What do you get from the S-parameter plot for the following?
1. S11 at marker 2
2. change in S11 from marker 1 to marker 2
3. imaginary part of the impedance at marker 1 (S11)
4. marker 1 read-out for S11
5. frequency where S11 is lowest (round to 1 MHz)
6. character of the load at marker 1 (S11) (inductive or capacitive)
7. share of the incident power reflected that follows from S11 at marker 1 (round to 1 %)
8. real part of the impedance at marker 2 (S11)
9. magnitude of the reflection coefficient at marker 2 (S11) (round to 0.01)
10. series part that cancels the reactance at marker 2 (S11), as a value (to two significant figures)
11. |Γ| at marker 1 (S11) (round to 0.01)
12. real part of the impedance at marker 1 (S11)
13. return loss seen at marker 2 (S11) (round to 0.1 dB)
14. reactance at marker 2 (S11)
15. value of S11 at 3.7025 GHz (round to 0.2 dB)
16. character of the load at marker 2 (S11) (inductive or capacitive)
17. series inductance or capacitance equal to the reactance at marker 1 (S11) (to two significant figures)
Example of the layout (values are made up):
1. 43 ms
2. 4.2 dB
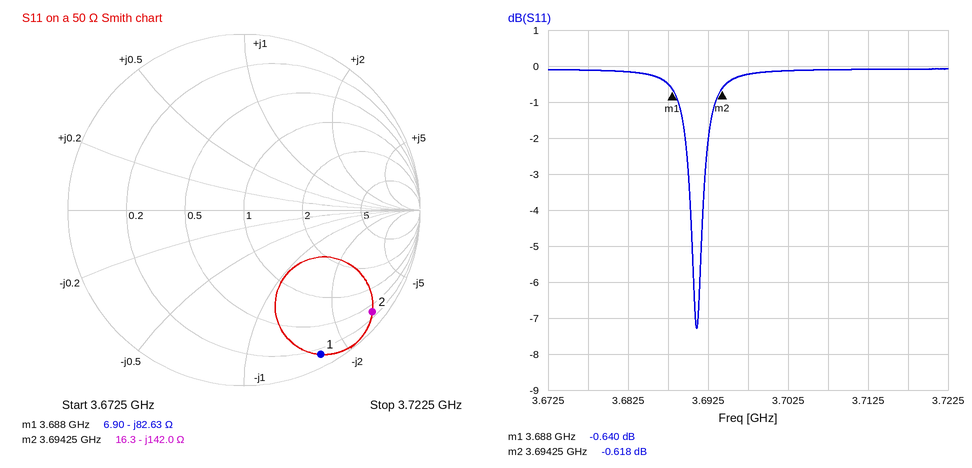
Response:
1. -0.618 dB
2. 0.022 dB
3. -82.63 Ω
4. -0.640 dB
5. 3.691 GHz
6. capacitive
7. 86 %
8. 16.3 Ω
9. 0.93
10. 6.1 nH
11. 0.93
12. 6.90 Ω
13. 0.6 dB
14. -142.0 Ω
15. -0.2 dB
16. capacitive
17. 520 fF
